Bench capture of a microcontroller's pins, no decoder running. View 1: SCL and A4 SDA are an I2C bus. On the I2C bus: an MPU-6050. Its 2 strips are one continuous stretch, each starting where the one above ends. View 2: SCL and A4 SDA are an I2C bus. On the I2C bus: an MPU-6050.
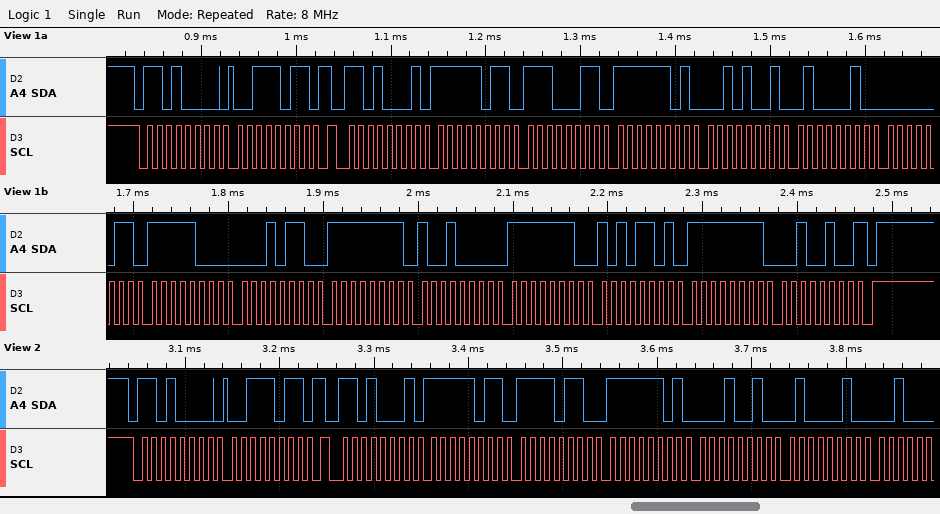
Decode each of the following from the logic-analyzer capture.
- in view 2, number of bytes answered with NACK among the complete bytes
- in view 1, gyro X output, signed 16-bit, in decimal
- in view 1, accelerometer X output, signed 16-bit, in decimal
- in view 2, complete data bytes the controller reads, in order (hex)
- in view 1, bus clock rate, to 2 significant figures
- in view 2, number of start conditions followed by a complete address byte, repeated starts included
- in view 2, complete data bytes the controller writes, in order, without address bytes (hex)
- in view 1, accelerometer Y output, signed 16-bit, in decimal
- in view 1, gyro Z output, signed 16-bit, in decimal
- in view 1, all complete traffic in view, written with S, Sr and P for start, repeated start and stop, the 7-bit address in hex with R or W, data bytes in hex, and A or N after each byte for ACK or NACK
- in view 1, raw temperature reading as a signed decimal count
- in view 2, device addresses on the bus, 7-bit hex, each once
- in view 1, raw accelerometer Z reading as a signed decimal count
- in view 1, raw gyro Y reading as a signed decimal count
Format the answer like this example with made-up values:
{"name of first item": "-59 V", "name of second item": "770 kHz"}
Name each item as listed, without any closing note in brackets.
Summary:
{"in view 2, number of bytes answered with NACK among the complete bytes": "0", "in view 1, gyro X output, signed 16-bit, in decimal": "-112", "in view 1, accelerometer X output, signed 16-bit, in decimal": "-1053", "in view 2, complete data bytes the controller reads, in order": "FB F6 FD 12 42", "in view 1, bus clock rate, to 2 significant figures": "100 kHz", "in view 2, number of start conditions followed by a complete address byte, repeated starts included": "2", "in view 2, complete data bytes the controller writes, in order, without address bytes": "3B", "in view 1, accelerometer Y output, signed 16-bit, in decimal": "-727", "in view 1, gyro Z output, signed 16-bit, in decimal": "-220", "in view 1, all complete traffic in view, written with S, Sr and P for start, repeated start and stop, the 7-bit address in hex with R or W, data bytes in hex, and A or N after each byte for ACK or NACK": "S 68W A 3B A Sr 68R A FB A E3 A FD A 29 A 42 A 03 A F8 A 16 A FF A 90 A FE A AD A FF A 24 N P", "in view 1, raw temperature reading as a signed decimal count": "-2026", "in view 2, device addresses on the bus, 7-bit hex, each once": "0x68", "in view 1, raw accelerometer Z reading as a signed decimal count": "16899", "in view 1, raw gyro Y reading as a signed decimal count": "-339"}
